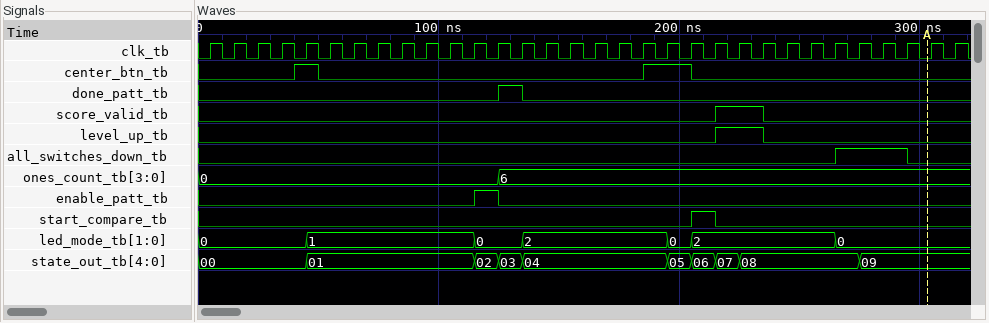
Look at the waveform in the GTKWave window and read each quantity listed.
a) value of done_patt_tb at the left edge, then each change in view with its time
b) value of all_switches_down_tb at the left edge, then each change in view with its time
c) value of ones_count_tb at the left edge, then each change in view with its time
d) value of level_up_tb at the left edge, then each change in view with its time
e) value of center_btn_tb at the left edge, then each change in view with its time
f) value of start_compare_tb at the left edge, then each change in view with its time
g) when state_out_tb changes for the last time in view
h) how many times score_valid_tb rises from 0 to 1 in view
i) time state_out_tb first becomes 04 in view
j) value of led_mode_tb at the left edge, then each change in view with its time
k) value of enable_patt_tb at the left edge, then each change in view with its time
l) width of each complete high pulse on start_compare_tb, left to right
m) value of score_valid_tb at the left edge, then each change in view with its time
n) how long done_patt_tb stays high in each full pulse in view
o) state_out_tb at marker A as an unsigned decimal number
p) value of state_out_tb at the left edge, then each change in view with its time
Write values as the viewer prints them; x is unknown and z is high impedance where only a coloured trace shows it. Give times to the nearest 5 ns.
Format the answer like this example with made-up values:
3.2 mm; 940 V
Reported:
0, 1 at 125 ns, 0 at 135 ns; 0, 1 at 265 ns, 0 at 295 ns; 0, 6 at 125 ns; 0, 1 at 215 ns, 0 at 235 ns; 0, 1 at 40 ns, 0 at 50 ns, 1 at 185 ns, 0 at 205 ns; 0, 1 at 205 ns, 0 at 215 ns; 275 ns; 1; 135 ns; 0, 1 at 45 ns, 0 at 115 ns, 2 at 135 ns, 0 at 195 ns, 2 at 205 ns, 0 at 265 ns; 0, 1 at 115 ns, 0 at 125 ns; 10 ns; 0, 1 at 215 ns, 0 at 235 ns; 10 ns; 9; 00, 01 at 45 ns, 02 at 115 ns, 03 at 125 ns, 04 at 135 ns, 05 at 195 ns, 06 at 205 ns, 07 at 215 ns, 08 at 225 ns, 09 at 275 ns
